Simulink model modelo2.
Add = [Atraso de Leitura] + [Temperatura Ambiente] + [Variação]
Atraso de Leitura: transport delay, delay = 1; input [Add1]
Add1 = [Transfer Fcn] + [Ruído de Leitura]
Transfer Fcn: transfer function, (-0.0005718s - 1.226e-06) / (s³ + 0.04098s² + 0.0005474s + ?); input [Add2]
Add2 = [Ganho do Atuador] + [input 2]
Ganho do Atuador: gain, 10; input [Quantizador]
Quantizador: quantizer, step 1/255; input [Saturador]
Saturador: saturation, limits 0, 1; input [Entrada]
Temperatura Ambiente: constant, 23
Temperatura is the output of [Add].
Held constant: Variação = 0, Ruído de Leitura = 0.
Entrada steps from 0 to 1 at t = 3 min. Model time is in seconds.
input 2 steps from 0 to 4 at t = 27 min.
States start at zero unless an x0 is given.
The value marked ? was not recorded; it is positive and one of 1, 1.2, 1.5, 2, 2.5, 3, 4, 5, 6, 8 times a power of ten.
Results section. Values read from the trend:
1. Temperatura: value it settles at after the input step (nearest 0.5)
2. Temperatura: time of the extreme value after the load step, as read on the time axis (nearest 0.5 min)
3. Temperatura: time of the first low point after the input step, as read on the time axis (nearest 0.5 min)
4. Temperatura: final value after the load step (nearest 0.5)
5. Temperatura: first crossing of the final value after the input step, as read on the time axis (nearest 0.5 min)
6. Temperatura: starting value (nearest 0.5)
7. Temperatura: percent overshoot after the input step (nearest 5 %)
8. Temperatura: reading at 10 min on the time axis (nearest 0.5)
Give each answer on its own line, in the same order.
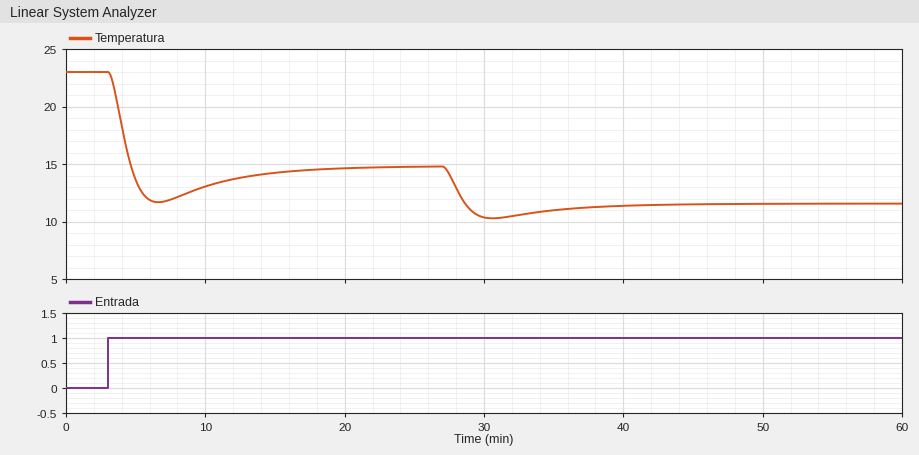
15.0
30.5 min
6.5 min
11.5
4.5 min
23.0
40 %
13.0
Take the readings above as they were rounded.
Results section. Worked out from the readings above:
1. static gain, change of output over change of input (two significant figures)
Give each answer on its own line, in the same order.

-8.0
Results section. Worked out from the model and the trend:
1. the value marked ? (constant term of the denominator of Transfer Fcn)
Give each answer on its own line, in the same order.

1.5e-06
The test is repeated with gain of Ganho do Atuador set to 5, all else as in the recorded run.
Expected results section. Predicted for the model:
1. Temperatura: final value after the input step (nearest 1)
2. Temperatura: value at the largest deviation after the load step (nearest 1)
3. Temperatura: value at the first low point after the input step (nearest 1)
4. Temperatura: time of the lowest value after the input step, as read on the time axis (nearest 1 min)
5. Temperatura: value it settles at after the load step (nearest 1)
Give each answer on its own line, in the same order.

19
14
17
7 min
16
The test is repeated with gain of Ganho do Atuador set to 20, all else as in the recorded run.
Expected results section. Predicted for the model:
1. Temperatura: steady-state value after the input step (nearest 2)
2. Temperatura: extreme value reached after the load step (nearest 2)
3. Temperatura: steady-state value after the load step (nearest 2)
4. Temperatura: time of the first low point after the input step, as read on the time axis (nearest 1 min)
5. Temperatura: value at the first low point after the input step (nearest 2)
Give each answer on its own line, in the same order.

6
2
4
7 min
0
